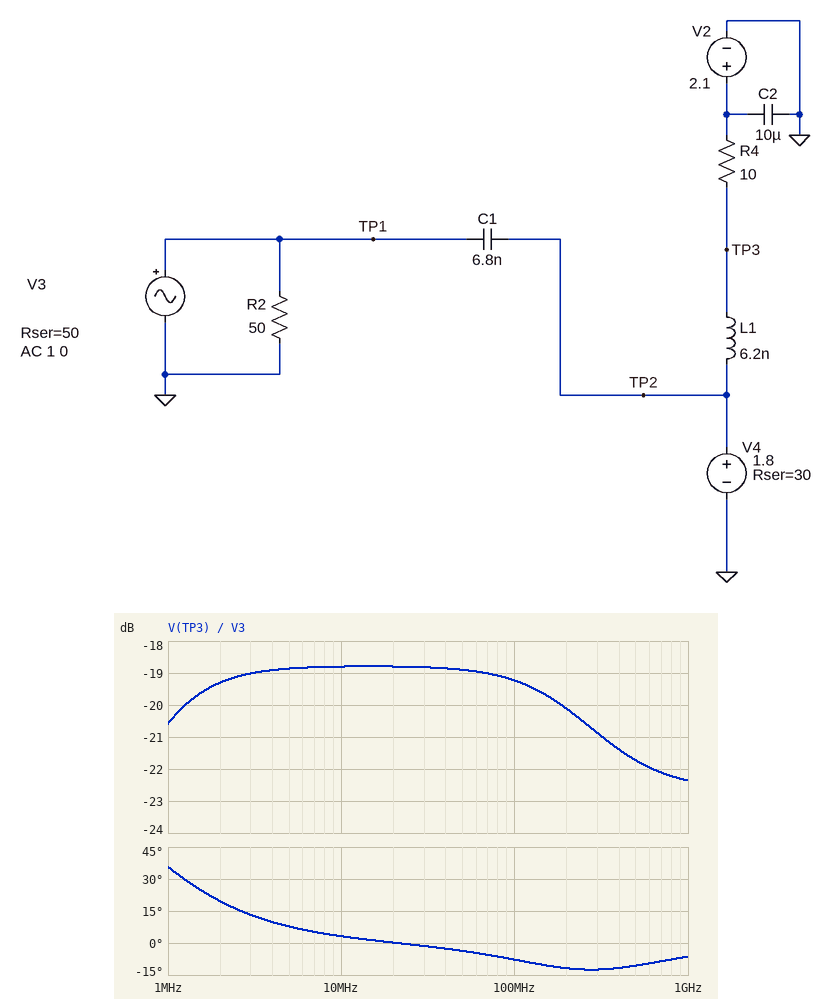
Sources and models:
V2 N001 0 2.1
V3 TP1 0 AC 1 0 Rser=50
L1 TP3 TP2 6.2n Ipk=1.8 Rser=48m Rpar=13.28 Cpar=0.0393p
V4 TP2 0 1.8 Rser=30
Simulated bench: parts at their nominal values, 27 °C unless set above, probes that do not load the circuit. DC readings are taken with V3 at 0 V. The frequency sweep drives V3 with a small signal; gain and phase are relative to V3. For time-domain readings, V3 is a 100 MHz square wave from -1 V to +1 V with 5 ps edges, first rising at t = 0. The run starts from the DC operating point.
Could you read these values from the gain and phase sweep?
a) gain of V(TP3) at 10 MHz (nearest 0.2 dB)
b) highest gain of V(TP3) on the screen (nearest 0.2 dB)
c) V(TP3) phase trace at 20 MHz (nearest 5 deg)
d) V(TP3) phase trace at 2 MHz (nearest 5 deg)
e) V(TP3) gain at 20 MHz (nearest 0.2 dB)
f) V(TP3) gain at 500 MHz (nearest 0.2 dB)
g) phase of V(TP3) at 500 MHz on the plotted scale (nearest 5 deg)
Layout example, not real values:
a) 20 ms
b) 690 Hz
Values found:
a) -18.8 dB
b) -18.8 dB
c) 0 deg
d) 20 deg
e) -18.8 dB
f) -21.8 dB
g) -10 deg
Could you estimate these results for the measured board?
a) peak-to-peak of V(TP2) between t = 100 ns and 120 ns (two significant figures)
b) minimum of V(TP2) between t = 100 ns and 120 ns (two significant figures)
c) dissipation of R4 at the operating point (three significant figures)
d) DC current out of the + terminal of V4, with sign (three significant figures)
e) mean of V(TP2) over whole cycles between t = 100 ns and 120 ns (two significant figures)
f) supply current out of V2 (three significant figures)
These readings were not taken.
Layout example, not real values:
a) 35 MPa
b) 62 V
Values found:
a) 460 mV
b) 1.9 V
c) 561 µW
d) -7.49 mA
e) 2.1 V
f) 7.49 mA
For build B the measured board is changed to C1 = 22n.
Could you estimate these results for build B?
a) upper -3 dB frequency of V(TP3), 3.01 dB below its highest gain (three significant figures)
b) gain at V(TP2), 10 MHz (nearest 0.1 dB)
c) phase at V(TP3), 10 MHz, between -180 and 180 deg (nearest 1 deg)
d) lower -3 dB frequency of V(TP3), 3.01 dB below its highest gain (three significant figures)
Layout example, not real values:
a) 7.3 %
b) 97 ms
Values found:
a) 523 MHz
b) -18.7 dB
c) 0 deg
d) 222 kHz
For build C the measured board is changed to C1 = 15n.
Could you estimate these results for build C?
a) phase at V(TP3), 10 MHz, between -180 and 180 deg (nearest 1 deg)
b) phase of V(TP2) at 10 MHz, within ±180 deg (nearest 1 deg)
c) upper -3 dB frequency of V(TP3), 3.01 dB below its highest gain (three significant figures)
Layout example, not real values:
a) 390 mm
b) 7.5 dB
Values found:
a) 1 deg
b) 3 deg
c) 524 MHz
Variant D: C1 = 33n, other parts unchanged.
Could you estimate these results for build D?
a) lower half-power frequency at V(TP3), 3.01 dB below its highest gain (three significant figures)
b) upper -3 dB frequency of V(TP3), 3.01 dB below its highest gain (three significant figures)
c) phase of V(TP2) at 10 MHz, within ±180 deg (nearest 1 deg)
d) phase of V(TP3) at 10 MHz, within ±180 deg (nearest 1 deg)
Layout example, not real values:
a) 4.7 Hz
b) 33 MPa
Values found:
a) 148 kHz
b) 522 MHz
c) 2 deg
d) 0 deg
